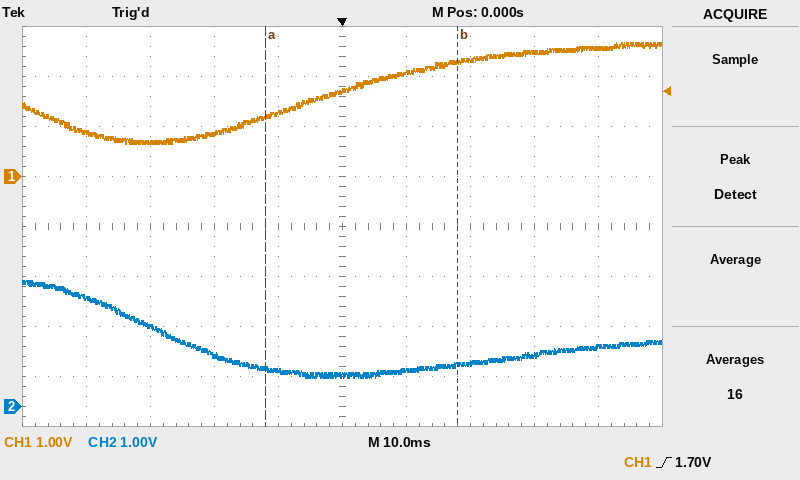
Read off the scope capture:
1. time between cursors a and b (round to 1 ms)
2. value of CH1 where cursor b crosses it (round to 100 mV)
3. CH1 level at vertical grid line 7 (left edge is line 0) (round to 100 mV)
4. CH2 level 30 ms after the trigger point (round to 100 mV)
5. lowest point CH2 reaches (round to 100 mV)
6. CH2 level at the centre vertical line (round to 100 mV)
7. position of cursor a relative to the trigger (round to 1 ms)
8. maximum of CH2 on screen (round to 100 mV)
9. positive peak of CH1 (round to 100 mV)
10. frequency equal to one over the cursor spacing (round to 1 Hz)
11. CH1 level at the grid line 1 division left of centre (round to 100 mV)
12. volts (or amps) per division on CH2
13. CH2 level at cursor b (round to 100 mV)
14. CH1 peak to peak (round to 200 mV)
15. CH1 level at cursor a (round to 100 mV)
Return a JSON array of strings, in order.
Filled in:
["30 ms", "2.3 V", "2.3 V", "1.0 V", "600 mV", "600 mV", "-12 ms", "2.5 V", "2.7 V", "33 Hz", "1.3 V", "1 V", "800 mV", "2.0 V", "1.2 V"]
